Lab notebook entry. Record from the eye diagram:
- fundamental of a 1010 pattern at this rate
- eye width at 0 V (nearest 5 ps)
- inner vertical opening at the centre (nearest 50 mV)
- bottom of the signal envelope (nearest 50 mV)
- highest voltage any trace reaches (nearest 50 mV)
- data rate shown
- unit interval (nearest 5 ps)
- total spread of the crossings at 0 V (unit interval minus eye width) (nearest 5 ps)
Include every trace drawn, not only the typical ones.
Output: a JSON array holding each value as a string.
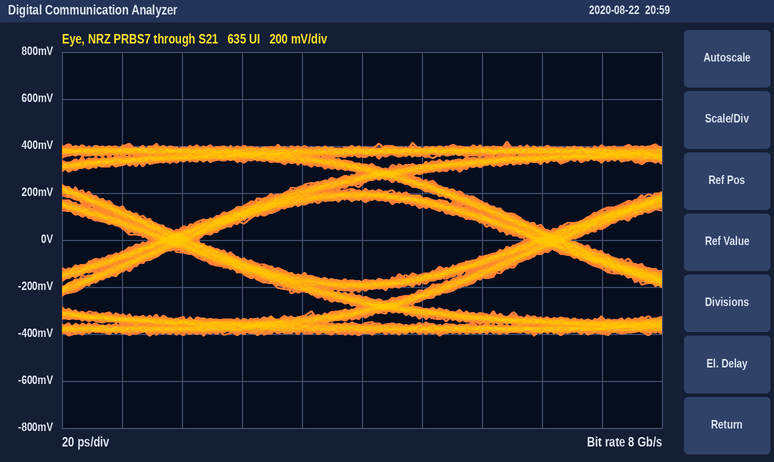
["4 GHz", "110 ps", "350 mV", "-400 mV", "400 mV", "8 Gb/s", "125 ps", "15 ps"]
